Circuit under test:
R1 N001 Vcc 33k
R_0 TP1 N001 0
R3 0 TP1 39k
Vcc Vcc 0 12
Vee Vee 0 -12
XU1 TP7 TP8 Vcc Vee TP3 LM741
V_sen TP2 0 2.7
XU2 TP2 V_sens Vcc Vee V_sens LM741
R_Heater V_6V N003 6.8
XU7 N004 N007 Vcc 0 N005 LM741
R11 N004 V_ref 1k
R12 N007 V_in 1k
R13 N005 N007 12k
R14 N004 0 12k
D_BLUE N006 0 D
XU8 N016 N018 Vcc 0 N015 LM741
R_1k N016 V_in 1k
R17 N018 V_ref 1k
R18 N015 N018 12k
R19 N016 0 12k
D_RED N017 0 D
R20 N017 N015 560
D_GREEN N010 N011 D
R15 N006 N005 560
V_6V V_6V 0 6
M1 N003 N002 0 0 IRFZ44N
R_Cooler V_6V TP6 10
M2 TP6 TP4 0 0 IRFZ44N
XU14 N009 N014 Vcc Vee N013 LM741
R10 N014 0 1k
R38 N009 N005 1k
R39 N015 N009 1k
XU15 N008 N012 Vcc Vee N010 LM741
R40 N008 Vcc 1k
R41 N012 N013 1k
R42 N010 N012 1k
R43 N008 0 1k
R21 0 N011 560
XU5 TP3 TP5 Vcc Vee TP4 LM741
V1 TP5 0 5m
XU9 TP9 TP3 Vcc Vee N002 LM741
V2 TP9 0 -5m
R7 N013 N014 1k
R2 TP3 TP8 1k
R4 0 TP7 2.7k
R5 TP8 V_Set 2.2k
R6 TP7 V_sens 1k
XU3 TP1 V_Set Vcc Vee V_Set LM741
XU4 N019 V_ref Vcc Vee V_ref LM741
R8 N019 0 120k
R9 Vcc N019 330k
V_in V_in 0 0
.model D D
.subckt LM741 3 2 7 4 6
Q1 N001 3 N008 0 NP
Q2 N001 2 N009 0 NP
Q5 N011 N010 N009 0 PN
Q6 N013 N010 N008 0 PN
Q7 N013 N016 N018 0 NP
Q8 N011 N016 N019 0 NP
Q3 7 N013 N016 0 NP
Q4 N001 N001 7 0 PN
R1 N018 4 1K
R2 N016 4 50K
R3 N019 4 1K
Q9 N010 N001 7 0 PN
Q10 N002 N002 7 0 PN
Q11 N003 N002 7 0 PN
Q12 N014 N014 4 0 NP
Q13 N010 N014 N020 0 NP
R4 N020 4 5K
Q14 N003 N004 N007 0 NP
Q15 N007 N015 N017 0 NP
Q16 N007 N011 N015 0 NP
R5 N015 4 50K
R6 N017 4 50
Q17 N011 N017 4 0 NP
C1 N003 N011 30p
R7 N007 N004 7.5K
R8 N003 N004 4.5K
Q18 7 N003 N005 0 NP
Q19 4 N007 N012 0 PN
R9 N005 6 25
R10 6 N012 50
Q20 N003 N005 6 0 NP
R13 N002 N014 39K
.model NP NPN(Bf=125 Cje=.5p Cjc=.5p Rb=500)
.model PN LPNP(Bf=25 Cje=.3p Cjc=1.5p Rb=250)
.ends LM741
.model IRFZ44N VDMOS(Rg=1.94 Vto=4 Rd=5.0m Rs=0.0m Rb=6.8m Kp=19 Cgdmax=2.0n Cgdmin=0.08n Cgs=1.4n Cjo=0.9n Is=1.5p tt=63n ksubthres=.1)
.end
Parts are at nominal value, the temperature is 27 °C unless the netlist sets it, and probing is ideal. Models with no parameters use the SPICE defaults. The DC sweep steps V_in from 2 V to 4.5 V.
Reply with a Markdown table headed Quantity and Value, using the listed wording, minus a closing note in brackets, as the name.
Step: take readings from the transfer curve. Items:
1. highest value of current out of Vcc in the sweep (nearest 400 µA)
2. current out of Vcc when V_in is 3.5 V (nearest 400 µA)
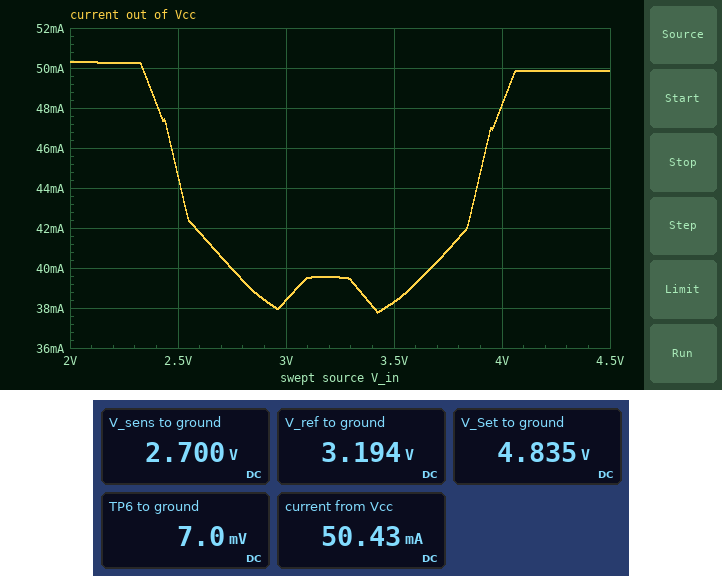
| Quantity | Value |
|---|---|
| highest value of current out of Vcc in the sweep | 50.4 mA |
| current out of Vcc when V_in is 3.5 V | 38.4 mA |
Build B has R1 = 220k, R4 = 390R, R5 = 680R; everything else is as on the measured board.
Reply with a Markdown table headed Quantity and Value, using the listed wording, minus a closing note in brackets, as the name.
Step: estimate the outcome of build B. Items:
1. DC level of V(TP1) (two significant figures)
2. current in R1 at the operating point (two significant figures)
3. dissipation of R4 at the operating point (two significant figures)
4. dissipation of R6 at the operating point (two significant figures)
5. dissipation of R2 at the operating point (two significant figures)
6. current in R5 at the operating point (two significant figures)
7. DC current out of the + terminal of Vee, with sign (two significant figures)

| Quantity | Value |
|---|---|
| DC level of V(TP1) | 720 mV |
| current in R1 at the operating point | 51 µA |
| dissipation of R4 at the operating point | 1.5 mW |
| dissipation of R6 at the operating point | 3.8 mW |
| dissipation of R2 at the operating point | 2.4 µW |
| current in R5 at the operating point | 49 µA |
| DC current out of the + terminal of Vee, with sign | -12 mA |
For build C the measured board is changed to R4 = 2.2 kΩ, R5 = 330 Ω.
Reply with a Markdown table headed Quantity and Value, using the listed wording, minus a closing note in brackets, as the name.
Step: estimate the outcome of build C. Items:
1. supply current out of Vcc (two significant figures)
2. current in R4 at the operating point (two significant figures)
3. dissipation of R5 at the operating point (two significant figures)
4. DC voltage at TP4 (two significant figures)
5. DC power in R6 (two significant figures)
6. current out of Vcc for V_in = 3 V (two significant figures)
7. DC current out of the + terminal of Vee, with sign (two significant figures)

| Quantity | Value |
|---|---|
| supply current out of Vcc | 58 mA |
| current in R4 at the operating point | 840 µA |
| dissipation of R5 at the operating point | 27 mW |
| DC voltage at TP4 | -11 V |
| DC power in R6 | 710 µW |
| current out of Vcc for V_in = 3 V | 46 mA |
| DC current out of the + terminal of Vee, with sign | -21 mA |
